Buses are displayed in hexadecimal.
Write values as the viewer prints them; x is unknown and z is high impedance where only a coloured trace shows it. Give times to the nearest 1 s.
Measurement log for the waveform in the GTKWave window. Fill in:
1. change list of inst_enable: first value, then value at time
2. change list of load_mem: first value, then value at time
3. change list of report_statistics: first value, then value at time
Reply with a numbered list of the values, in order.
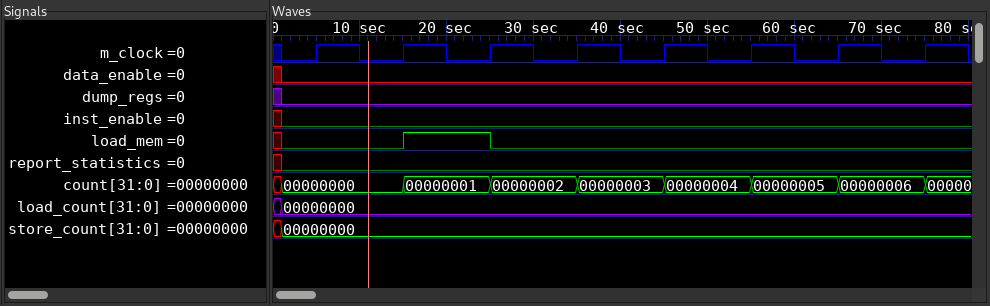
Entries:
1. x, 0 at 1 s
2. x, 0 at 1 s, 1 at 15 s, 0 at 25 s
3. x, 0 at 1 s
